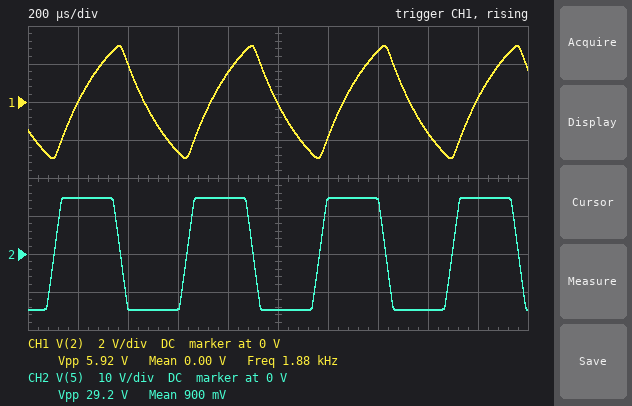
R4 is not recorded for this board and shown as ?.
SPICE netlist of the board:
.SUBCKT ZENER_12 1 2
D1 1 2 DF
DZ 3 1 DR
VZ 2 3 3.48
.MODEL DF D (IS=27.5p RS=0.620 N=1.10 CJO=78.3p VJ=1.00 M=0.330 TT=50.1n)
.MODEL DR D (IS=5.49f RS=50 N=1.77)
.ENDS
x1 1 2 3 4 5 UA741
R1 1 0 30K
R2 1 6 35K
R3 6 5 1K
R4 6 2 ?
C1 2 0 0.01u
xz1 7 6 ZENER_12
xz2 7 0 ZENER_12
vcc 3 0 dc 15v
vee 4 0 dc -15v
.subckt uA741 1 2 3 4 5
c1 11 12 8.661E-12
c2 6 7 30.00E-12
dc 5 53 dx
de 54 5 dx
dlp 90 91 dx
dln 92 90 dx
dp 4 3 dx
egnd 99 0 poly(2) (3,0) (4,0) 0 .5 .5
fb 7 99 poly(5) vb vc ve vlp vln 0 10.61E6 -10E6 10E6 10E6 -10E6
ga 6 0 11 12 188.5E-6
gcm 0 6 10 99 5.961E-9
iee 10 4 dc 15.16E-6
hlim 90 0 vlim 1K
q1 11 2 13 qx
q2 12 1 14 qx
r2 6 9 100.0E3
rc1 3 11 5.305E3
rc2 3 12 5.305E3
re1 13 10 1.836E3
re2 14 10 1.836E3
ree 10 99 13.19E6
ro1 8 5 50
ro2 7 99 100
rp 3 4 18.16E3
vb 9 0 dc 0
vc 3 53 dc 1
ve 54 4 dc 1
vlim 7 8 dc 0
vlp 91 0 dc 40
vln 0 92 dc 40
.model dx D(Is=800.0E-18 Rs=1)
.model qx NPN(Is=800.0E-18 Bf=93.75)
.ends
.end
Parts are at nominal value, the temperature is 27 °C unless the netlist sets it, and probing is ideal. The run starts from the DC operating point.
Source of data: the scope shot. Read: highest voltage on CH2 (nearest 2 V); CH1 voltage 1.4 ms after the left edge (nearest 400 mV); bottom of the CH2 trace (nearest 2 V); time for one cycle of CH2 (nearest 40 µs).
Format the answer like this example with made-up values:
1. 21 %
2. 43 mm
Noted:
1. 14 V
2. 2.8 V
3. -14 V
4. 520 µs
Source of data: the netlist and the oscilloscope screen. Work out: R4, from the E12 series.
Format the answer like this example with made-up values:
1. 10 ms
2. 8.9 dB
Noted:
1. 22 kΩ
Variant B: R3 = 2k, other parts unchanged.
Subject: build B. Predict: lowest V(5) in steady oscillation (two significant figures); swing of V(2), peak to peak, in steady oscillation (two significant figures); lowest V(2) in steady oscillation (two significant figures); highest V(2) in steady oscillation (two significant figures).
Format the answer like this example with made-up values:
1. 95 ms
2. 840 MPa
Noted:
1. -15 V
2. 5.7 V
3. -2.8 V
4. 2.8 V
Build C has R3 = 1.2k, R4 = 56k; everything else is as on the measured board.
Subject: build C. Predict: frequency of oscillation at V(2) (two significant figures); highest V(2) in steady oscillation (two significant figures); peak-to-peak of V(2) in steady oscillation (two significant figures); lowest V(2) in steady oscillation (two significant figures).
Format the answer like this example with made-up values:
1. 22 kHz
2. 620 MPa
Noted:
1. 820 Hz
2. 2.8 V
3. 5.5 V
4. -2.8 V
